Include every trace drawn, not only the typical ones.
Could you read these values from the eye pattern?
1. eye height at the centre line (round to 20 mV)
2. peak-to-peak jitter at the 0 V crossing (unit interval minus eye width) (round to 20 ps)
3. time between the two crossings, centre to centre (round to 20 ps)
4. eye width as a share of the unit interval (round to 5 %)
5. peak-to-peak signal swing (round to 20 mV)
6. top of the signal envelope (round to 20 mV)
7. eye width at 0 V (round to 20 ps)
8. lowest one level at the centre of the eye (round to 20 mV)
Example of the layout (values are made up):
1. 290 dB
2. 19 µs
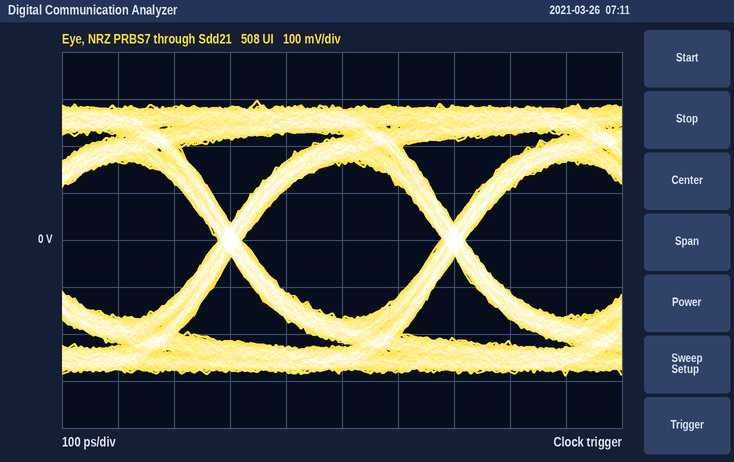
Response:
1. 340 mV
2. 40 ps
3. 400 ps
4. 90 %
5. 580 mV
6. 300 mV
7. 360 ps
8. 160 mV
